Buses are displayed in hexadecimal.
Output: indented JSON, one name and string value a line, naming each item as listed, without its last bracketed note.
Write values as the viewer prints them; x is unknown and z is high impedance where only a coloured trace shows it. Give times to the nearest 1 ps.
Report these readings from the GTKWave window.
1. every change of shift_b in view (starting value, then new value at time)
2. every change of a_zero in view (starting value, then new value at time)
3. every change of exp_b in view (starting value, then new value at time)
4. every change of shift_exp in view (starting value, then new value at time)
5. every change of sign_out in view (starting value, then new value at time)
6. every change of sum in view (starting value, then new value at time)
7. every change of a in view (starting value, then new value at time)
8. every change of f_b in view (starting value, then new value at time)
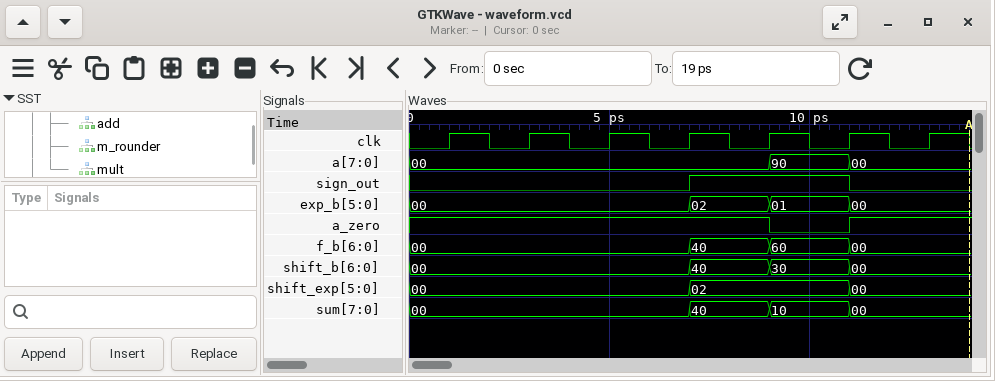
{
  "every change of shift_b in view": "00, 40 at 7 ps, 30 at 9 ps, 00 at 11 ps",
  "every change of a_zero in view": "1, 0 at 9 ps, 1 at 11 ps",
  "every change of exp_b in view": "00, 02 at 7 ps, 01 at 9 ps, 00 at 11 ps",
  "every change of shift_exp in view": "00, 02 at 7 ps, 00 at 11 ps",
  "every change of sign_out in view": "0, 1 at 7 ps, 0 at 11 ps",
  "every change of sum in view": "00, 40 at 7 ps, 10 at 9 ps, 00 at 11 ps",
  "every change of a in view": "00, 90 at 9 ps, 00 at 11 ps",
  "every change of f_b in view": "00, 40 at 7 ps, 60 at 9 ps, 00 at 11 ps"
}
